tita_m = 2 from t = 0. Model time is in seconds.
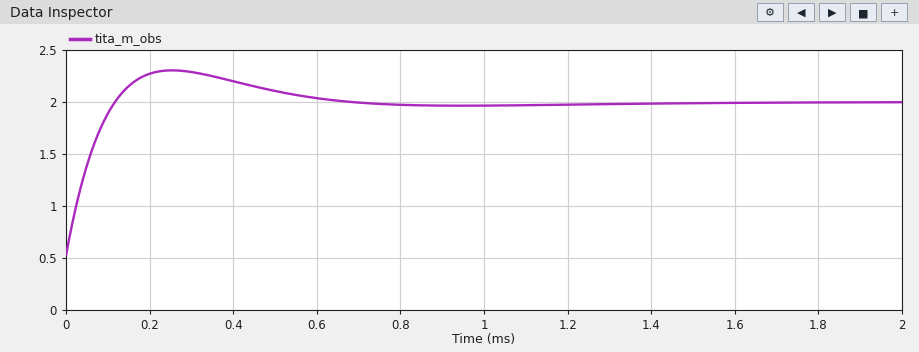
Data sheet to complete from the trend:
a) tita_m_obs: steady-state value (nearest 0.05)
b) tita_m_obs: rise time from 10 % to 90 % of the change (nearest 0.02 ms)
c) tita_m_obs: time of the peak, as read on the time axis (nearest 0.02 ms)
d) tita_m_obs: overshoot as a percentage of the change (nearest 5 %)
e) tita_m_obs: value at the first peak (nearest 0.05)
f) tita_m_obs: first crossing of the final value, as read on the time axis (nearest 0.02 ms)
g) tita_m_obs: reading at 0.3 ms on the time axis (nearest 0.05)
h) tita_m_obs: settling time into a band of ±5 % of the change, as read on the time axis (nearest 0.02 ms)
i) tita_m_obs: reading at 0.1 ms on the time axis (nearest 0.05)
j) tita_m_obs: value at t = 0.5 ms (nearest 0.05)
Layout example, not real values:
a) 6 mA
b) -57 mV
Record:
a) 2.00
b) 0.08 ms
c) 0.26 ms
d) 20 %
e) 2.30
f) 0.12 ms
g) 2.30
h) 0.54 ms
i) 1.90
j) 2.10
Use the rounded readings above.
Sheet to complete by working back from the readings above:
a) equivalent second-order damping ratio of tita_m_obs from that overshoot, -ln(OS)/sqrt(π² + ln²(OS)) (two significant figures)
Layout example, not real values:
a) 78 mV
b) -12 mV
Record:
a) 0.46
